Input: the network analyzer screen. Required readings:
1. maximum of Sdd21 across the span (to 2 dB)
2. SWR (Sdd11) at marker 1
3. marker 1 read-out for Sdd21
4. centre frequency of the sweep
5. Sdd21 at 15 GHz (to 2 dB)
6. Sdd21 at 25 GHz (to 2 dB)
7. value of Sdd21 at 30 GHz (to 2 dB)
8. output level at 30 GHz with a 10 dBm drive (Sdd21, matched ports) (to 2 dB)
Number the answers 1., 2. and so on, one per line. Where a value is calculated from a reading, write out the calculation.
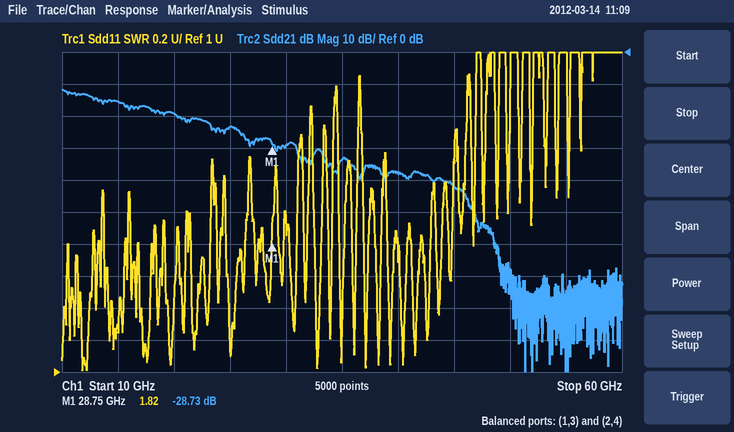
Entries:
1. -12 dB
2. 1.82
3. -28.73 dB
4. 35 GHz
5. -16 dB
6. -24 dB
7. -30 dB
8. 10 dBm + (-30 dB) = -20 dBm
